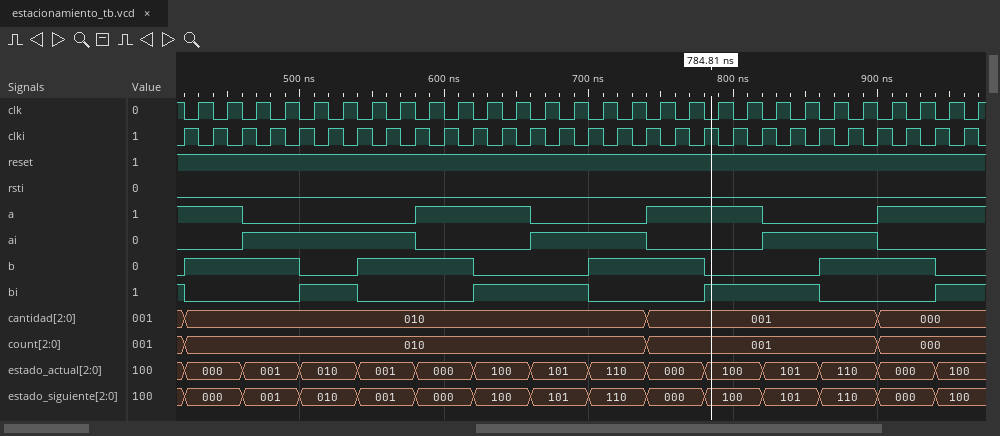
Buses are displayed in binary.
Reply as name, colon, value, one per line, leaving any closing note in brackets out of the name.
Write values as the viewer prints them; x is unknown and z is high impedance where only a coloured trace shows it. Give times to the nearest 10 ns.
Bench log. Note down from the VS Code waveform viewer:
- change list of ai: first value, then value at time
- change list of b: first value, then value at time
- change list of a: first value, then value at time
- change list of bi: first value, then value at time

change list of ai: first value, then value at time: 0, 1 at 460 ns, 0 at 580 ns, 1 at 660 ns, 0 at 740 ns, 1 at 820 ns, 0 at 900 ns
change list of b: first value, then value at time: 0, 1 at 420 ns, 0 at 500 ns, 1 at 540 ns, 0 at 620 ns, 1 at 700 ns, 0 at 780 ns, 1 at 860 ns, 0 at 940 ns
change list of a: first value, then value at time: 1, 0 at 460 ns, 1 at 580 ns, 0 at 660 ns, 1 at 740 ns, 0 at 820 ns, 1 at 900 ns
change list of bi: first value, then value at time: 1, 0 at 420 ns, 1 at 500 ns, 0 at 540 ns, 1 at 620 ns, 0 at 700 ns, 1 at 780 ns, 0 at 860 ns, 1 at 940 ns
